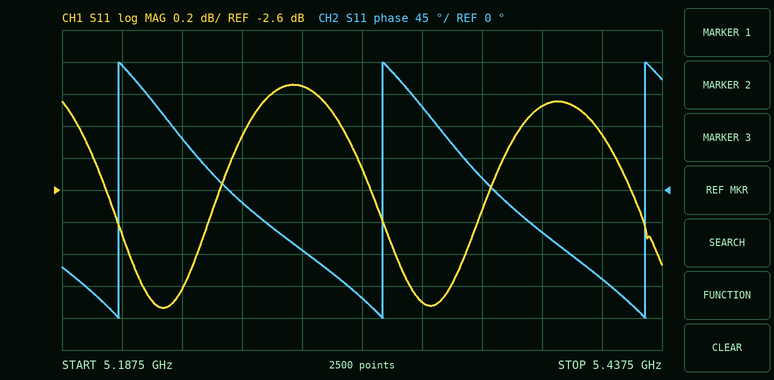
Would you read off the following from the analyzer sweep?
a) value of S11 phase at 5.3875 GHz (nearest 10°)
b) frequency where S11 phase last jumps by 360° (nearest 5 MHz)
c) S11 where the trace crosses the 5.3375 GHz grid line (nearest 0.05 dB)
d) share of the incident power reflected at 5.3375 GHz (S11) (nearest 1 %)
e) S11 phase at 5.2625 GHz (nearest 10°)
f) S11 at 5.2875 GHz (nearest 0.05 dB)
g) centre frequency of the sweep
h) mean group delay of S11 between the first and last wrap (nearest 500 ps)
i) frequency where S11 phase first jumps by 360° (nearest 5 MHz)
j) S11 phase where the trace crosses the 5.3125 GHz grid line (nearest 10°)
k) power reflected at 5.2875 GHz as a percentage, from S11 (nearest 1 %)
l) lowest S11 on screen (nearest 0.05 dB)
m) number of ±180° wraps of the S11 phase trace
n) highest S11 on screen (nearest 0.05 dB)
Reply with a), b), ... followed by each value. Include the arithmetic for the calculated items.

a) -60°
b) 5.430 GHz
c) -3.30 dB
d) 10^(-3.3/10) ≈ 47 %
e) -20°
f) -1.95 dB
g) 5.3125 GHz
h) 2 cycles / (5.430 GHz − 5.210 GHz) ≈ 9.09 ns, so 9.0 ns to the nearest 500 ps
i) 5.210 GHz
j) -150°
k) 10^(-1.95/10) ≈ 64 %
l) -3.35 dB
m) 3
n) -1.95 dB
